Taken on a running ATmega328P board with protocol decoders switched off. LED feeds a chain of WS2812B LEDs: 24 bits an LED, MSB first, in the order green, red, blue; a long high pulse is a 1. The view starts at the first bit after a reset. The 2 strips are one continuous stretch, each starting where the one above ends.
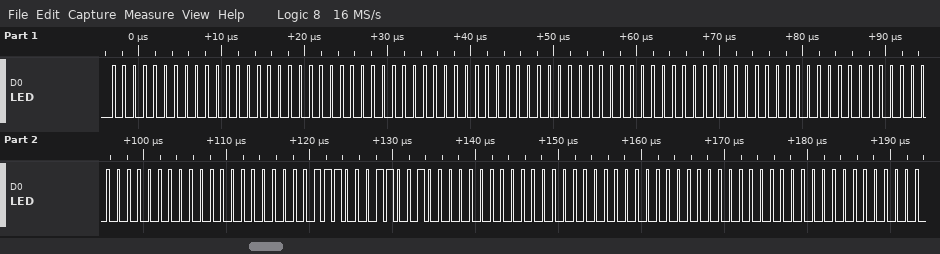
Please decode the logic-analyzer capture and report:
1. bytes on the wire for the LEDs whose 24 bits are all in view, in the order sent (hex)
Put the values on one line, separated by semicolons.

00 00 00 00 00 00 00 00 00 00 00 00 1C 64 00 00 00 00
